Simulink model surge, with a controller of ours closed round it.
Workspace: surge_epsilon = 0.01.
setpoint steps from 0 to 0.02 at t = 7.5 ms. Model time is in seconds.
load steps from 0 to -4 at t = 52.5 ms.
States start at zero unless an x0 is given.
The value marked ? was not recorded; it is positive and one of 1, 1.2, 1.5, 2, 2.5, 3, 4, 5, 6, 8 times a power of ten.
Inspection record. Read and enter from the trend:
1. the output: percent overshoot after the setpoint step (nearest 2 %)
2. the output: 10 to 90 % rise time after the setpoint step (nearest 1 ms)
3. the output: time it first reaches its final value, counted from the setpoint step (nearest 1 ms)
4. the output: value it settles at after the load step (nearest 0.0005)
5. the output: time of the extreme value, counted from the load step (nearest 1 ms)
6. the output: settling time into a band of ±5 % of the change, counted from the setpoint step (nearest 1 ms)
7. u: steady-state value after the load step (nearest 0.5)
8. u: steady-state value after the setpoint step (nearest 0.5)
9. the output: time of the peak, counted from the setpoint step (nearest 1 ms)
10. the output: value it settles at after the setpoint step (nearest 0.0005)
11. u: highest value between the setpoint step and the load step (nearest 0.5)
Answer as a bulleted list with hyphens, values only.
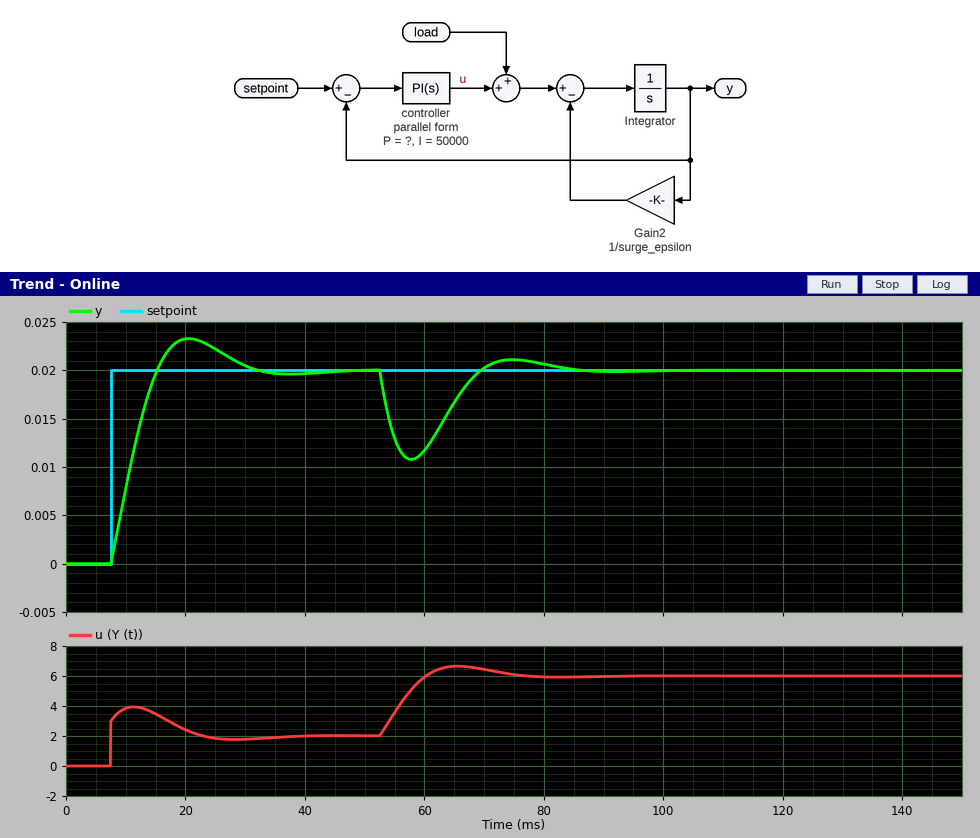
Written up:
- 16 %
- 6 ms
- 8 ms
- 0.0200
- 5 ms
- 21 ms
- 6.0
- 2.0
- 13 ms
- 0.0200
- 4.0
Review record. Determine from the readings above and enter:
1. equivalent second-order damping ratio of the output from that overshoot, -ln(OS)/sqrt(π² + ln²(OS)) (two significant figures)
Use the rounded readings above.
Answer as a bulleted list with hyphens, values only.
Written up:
- 0.50
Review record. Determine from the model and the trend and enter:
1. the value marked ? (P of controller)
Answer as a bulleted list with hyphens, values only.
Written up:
- 150
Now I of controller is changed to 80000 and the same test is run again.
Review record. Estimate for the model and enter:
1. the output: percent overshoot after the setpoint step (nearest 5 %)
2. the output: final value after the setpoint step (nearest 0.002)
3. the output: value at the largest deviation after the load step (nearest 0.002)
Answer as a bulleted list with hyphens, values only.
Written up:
- 25 %
- 0.020
- 0.012
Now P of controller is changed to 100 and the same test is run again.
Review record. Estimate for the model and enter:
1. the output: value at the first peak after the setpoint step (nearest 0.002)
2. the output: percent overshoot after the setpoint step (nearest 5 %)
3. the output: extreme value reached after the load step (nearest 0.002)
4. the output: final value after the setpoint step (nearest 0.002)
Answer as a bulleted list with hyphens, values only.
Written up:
- 0.024
- 25 %
- 0.010
- 0.020
